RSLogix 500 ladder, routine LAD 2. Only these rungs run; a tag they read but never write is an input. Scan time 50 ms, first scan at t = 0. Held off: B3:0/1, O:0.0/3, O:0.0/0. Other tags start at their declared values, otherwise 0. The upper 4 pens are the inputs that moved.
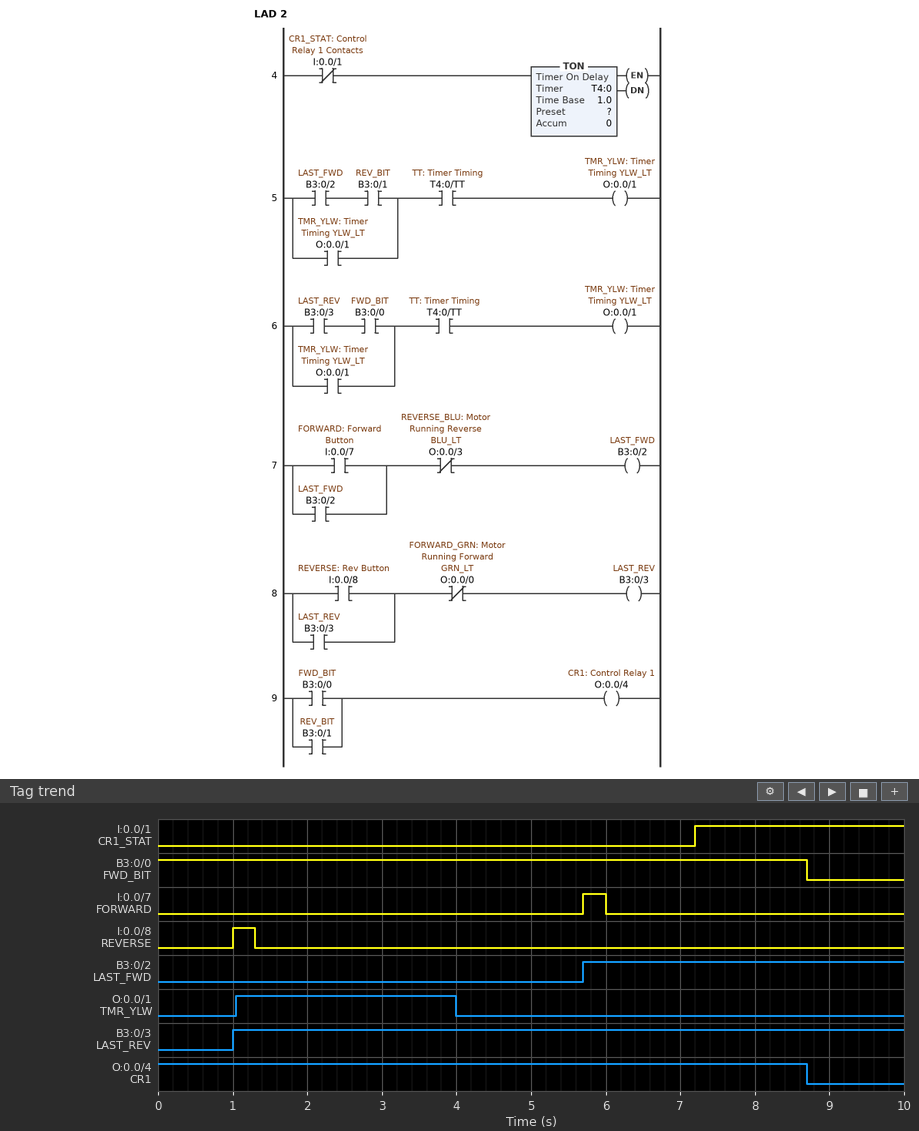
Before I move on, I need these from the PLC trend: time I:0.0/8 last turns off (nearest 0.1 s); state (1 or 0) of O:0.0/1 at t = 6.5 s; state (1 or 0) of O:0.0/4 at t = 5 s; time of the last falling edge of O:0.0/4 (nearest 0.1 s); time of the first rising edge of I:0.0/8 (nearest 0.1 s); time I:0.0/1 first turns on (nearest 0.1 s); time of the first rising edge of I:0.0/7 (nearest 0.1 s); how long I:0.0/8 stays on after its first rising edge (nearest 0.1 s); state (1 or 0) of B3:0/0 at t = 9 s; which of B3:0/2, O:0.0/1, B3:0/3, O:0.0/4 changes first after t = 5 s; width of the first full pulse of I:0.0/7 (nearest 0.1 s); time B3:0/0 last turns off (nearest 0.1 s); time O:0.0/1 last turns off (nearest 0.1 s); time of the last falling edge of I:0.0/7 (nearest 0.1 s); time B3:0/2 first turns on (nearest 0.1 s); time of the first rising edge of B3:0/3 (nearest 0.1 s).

1.3 s
0
1
8.7 s
1.0 s
7.2 s
5.7 s
0.3 s
0
B3:0/2
0.3 s
8.7 s
4.0 s
6.0 s
5.7 s
1.0 s
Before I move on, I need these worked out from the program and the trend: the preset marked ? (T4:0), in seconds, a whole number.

4 s
